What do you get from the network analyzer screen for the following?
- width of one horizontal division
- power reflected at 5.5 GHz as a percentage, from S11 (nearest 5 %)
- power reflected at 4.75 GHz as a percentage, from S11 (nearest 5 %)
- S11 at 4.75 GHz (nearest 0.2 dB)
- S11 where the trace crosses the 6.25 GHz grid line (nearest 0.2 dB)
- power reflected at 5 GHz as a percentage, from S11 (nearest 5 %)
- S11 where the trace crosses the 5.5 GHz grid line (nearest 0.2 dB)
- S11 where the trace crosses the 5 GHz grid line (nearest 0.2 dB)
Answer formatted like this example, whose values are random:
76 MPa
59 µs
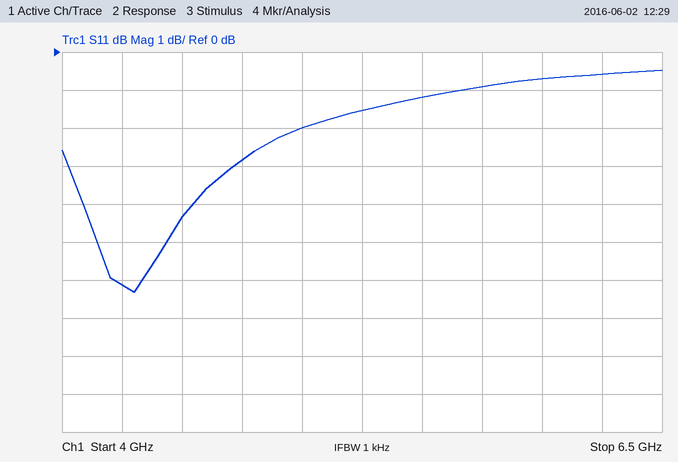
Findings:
250 MHz
75 %
50 %
-2.8 dB
-0.6 dB
65 %
-1.2 dB
-2.0 dB
